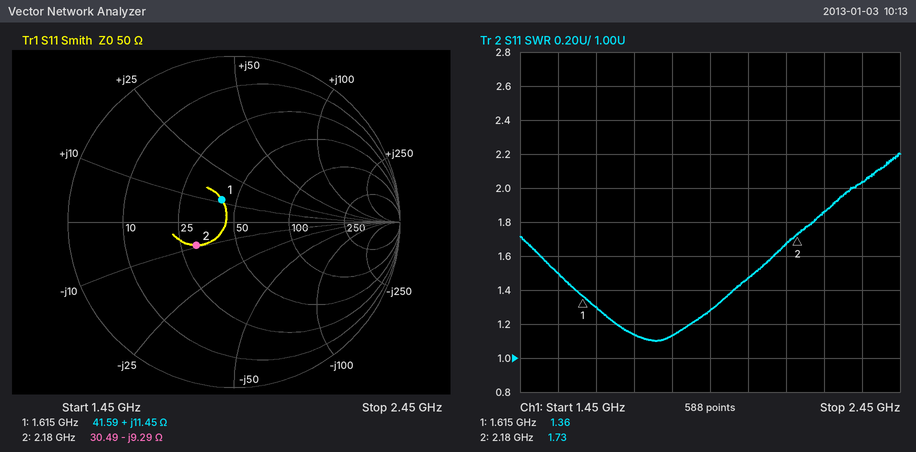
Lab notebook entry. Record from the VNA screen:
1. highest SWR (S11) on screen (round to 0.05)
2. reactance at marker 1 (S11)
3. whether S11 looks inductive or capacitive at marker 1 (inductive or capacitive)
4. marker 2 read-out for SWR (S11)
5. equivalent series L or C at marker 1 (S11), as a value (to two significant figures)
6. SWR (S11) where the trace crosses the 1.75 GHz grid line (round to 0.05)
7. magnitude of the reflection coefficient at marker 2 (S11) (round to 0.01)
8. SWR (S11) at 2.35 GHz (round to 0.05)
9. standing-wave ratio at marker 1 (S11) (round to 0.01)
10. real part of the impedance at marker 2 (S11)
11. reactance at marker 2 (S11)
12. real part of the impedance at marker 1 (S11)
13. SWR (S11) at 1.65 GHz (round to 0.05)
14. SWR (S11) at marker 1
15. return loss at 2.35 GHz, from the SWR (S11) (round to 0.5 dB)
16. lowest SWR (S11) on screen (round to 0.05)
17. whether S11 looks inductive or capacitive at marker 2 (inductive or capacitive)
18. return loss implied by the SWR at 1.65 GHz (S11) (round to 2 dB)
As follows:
2.20
+11.45 Ω
inductive
1.73
1.1 nH
1.15
0.27
2.05
1.36
30.49 Ω
-9.29 Ω
41.59 Ω
1.30
1.36
9.5 dB
1.10
capacitive
18 dB
